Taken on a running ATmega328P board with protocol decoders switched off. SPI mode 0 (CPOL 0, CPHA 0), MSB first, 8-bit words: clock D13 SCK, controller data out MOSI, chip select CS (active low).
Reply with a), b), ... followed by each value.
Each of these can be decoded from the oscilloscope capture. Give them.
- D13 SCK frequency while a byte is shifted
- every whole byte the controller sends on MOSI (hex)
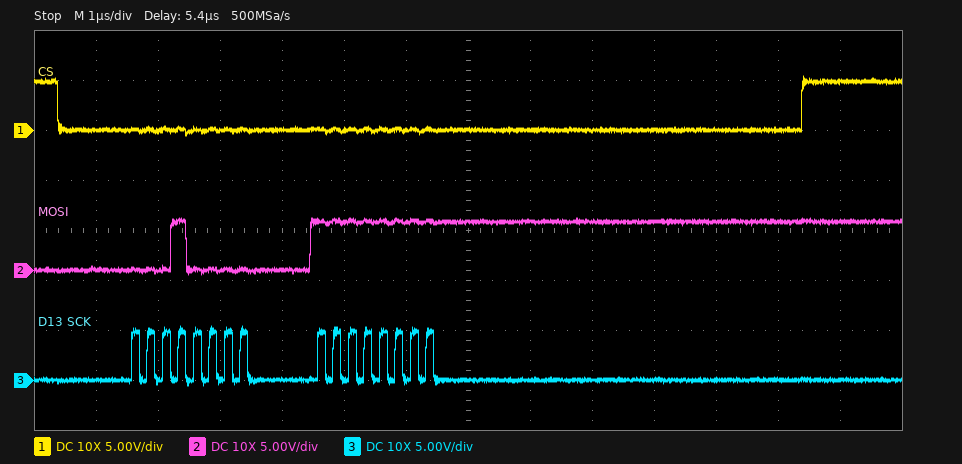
a) 4 MHz
b) 0x10 0xFF
